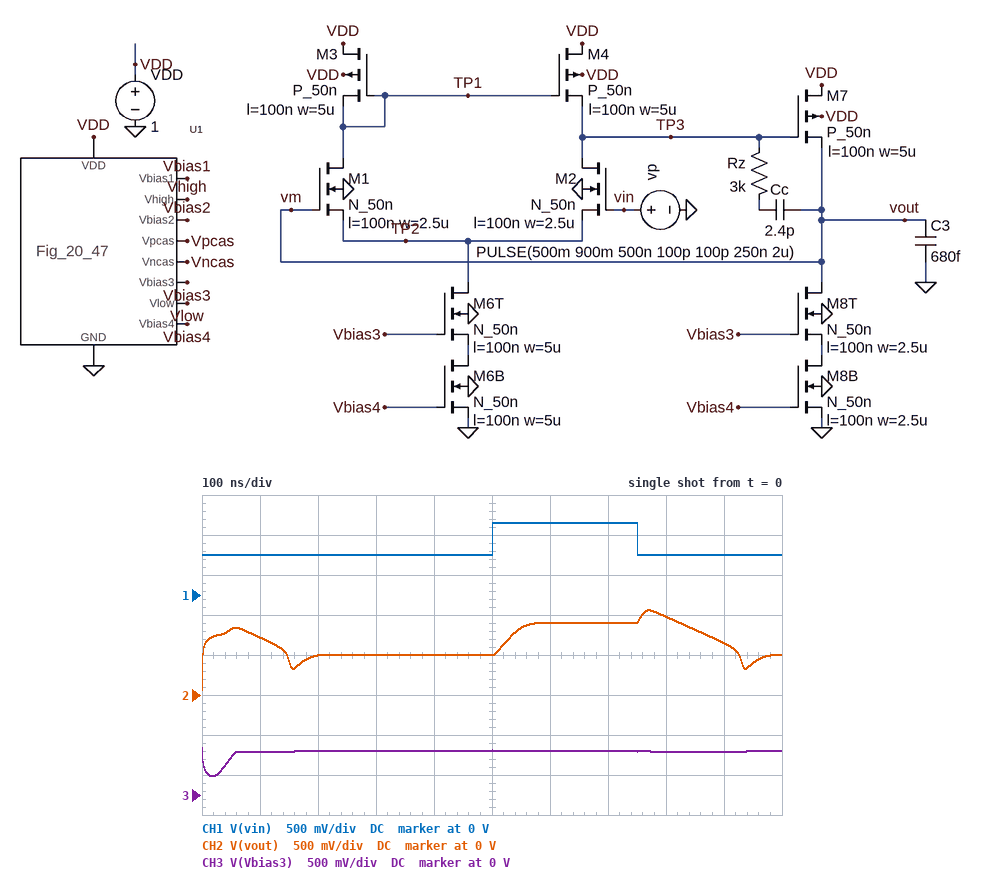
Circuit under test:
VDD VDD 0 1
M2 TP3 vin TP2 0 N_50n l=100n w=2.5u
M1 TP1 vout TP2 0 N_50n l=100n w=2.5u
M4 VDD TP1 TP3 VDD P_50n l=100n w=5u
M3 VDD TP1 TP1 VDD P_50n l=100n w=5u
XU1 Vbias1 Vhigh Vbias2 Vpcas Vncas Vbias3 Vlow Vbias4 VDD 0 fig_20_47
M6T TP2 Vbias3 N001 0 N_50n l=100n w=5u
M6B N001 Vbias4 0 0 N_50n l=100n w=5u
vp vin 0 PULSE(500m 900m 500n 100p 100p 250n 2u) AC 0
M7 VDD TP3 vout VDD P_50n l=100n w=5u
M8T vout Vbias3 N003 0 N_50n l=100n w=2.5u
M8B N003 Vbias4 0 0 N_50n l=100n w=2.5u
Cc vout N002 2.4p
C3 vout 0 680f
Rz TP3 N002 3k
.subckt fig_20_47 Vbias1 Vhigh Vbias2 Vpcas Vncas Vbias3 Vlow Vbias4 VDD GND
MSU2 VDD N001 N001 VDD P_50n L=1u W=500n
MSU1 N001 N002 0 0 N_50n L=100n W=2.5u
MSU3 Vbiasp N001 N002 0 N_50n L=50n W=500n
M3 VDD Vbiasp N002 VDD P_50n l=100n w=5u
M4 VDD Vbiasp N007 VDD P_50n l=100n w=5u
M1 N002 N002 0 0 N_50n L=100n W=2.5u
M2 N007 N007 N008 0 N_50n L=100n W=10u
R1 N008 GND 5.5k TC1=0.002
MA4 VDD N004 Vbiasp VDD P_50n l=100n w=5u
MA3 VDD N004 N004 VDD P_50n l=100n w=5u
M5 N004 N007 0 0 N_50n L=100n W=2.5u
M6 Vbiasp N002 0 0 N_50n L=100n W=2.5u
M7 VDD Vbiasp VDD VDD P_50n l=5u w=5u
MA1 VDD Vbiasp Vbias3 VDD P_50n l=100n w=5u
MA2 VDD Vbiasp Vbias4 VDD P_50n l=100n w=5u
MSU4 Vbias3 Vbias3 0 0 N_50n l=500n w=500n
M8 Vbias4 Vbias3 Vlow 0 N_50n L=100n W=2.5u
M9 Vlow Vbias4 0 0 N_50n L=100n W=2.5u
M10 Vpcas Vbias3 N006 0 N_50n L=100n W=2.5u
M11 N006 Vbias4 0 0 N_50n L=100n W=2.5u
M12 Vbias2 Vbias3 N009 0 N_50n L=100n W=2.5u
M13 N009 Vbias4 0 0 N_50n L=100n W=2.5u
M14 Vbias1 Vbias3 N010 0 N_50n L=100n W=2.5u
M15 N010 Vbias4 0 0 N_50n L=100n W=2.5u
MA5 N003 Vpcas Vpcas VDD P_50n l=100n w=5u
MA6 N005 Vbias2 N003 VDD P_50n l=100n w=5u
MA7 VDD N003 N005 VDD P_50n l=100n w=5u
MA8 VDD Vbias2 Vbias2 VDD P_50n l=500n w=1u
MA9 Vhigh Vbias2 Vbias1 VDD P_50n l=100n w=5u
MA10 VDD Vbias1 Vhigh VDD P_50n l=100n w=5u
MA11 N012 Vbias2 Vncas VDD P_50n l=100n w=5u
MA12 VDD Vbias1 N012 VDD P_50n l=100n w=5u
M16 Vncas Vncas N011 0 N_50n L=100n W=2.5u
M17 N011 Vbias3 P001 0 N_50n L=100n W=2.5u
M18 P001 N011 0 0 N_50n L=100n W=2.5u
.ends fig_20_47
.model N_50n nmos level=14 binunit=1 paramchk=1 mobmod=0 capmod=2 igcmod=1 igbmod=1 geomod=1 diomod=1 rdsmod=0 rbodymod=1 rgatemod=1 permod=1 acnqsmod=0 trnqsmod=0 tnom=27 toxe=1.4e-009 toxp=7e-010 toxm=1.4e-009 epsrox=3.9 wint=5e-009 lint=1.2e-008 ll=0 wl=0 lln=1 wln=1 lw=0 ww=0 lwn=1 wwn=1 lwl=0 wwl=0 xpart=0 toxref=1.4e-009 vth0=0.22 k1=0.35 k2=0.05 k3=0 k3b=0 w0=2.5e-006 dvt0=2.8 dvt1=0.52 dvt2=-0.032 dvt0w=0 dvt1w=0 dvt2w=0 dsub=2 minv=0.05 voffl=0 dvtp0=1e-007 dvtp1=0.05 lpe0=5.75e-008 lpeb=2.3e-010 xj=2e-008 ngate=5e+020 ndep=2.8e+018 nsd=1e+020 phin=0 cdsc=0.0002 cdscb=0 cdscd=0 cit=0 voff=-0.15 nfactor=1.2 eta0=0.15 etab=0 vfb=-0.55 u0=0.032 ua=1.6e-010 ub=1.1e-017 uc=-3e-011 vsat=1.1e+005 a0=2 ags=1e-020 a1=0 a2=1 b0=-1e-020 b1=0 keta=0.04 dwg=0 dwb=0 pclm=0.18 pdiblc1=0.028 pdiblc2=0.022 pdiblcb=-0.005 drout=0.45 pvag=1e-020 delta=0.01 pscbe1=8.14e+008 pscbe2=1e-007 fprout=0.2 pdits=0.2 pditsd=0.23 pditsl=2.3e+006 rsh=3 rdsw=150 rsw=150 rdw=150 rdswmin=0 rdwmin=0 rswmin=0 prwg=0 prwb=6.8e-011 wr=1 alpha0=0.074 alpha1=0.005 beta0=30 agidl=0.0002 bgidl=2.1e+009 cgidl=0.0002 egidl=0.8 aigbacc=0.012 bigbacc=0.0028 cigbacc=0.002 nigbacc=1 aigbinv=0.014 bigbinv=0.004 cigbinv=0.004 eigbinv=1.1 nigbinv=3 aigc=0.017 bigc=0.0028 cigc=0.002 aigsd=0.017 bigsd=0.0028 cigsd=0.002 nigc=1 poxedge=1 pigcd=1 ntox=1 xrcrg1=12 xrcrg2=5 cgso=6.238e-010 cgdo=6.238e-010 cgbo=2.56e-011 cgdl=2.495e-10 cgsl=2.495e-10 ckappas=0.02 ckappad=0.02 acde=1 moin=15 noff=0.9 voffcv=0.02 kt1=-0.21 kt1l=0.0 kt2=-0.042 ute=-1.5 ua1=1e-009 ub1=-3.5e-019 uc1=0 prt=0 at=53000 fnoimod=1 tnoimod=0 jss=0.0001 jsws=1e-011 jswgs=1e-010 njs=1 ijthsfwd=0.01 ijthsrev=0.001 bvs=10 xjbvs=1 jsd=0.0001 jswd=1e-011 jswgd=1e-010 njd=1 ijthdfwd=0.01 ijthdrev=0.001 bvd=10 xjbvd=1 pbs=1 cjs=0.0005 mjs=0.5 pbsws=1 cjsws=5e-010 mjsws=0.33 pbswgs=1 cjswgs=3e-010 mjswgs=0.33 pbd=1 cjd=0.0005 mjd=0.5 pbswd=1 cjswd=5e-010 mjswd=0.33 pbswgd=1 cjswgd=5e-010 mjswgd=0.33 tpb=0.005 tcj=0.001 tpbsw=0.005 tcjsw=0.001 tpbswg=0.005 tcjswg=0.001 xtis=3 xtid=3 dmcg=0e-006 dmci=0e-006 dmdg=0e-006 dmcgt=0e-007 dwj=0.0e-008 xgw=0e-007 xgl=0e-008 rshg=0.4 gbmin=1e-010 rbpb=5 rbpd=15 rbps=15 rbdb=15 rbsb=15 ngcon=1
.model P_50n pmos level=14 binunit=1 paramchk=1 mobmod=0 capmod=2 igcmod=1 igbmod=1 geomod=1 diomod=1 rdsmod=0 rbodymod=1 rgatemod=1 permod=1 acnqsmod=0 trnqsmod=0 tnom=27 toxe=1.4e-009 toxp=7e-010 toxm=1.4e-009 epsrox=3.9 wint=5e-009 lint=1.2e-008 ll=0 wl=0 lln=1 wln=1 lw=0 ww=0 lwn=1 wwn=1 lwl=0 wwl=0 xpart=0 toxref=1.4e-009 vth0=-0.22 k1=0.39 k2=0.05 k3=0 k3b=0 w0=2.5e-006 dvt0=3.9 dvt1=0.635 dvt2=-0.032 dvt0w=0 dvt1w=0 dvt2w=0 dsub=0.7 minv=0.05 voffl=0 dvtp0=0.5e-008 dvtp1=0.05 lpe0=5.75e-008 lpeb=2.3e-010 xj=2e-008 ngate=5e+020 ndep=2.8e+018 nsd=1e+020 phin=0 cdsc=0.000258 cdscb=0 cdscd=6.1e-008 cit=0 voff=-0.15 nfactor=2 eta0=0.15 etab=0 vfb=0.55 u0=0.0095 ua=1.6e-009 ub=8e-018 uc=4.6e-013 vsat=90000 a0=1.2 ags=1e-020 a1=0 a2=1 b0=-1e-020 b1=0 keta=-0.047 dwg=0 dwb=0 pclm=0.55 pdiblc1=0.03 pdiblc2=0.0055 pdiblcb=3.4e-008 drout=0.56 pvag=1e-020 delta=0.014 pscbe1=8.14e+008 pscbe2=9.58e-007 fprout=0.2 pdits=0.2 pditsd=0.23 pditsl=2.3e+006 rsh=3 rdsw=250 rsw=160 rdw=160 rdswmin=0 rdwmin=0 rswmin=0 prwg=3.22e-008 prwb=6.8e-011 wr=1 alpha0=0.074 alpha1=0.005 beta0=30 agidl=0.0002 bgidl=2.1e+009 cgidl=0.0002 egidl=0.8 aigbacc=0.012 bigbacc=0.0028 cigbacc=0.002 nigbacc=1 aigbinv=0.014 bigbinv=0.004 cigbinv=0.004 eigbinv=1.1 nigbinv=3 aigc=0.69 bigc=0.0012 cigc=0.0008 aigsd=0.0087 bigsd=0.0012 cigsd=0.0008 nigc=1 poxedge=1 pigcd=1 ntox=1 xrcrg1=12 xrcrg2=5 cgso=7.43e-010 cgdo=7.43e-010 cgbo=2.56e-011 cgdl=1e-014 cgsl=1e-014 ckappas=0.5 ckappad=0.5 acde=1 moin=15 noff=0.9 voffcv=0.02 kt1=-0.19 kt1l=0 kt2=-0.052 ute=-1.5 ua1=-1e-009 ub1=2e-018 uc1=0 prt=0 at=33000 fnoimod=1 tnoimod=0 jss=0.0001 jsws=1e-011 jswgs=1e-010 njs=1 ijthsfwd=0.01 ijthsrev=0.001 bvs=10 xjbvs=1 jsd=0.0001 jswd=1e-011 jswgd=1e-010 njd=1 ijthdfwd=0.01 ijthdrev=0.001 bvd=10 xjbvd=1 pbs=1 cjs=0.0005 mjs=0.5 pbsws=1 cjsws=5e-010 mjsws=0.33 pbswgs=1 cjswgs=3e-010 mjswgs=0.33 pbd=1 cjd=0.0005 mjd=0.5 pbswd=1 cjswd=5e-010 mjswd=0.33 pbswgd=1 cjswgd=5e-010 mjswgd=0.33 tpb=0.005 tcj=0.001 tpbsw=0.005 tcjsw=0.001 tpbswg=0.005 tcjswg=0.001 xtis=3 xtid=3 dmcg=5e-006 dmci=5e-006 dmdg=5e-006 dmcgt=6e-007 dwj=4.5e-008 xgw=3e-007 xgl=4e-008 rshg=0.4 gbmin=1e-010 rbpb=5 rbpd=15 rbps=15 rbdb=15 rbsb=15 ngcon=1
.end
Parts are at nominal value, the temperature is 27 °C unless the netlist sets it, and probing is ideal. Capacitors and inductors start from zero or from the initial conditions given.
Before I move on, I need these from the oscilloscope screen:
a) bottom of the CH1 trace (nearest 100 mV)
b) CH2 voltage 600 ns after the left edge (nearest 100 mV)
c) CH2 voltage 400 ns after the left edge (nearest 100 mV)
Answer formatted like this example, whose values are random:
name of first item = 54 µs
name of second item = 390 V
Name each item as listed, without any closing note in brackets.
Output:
bottom of the CH1 trace = 500 mV
CH2 voltage 600 ns after the left edge = 900 mV
CH2 voltage 400 ns after the left edge = 500 mV
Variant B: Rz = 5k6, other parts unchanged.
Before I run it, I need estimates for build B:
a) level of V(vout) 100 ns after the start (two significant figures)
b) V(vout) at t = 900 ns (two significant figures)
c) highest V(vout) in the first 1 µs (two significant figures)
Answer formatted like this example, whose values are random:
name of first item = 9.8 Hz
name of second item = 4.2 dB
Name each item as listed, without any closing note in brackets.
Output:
level of V(vout) 100 ns after the start = 700 mV
V(vout) at t = 900 ns = 630 mV
highest V(vout) in the first 1 µs = 1.0 V
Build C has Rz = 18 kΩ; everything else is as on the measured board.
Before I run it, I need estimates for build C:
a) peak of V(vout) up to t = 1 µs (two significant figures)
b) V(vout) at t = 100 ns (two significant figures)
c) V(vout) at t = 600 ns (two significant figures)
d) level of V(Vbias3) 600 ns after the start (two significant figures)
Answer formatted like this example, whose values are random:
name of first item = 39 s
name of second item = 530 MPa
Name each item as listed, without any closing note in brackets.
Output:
peak of V(vout) up to t = 1 µs = 950 mV
V(vout) at t = 100 ns = 630 mV
V(vout) at t = 600 ns = 880 mV
level of V(Vbias3) 600 ns after the start = 540 mV
